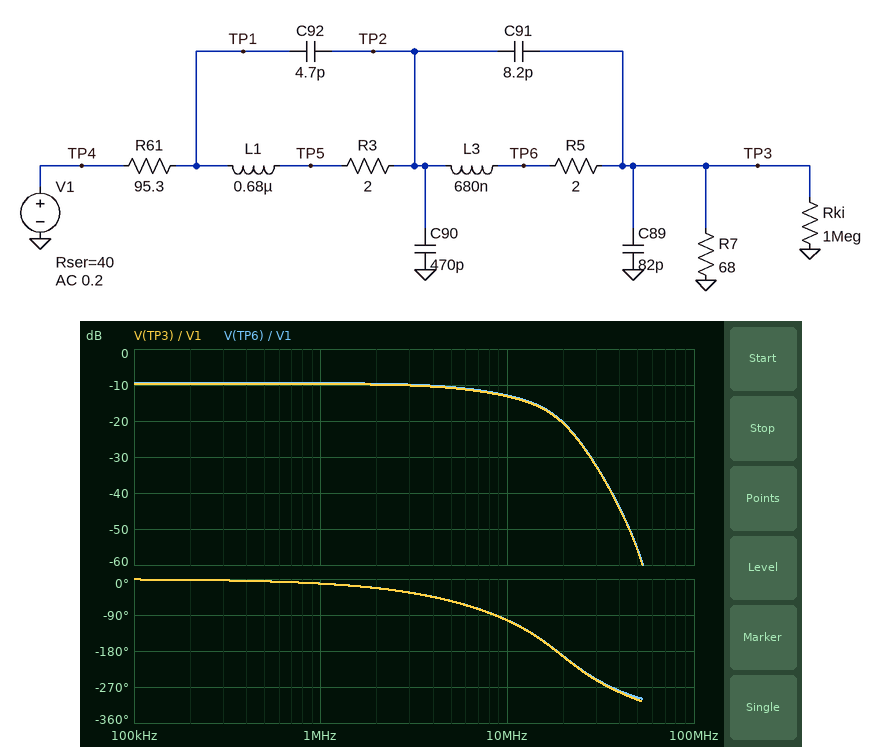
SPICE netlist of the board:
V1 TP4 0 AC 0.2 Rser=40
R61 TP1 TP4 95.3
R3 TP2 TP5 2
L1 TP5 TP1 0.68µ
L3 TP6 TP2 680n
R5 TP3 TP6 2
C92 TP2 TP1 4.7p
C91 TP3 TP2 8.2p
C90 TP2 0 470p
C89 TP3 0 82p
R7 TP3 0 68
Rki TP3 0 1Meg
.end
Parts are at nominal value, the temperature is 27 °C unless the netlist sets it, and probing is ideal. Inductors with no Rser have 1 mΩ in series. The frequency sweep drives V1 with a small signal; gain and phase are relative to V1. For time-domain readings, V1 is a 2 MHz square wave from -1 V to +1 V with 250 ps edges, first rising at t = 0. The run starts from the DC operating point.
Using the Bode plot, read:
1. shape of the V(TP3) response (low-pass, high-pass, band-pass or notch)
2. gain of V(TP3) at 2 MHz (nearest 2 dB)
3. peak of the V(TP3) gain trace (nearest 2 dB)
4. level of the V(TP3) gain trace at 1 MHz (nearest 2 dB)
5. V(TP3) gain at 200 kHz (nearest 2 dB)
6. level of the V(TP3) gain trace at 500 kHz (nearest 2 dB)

low-pass
-10 dB
-10 dB
-10 dB
-10 dB
-10 dB
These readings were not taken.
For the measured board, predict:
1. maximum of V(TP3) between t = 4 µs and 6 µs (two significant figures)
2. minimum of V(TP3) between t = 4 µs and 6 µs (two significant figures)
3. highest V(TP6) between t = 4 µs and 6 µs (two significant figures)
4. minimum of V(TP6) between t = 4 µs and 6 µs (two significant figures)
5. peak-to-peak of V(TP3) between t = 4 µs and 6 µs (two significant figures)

330 mV
-330 mV
340 mV
-340 mV
660 mV
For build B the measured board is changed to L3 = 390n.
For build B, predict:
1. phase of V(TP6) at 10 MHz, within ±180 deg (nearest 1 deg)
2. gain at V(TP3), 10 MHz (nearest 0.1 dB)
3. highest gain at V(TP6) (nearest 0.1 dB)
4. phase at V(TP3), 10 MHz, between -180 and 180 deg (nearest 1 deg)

-89 deg
-13.8 dB
-9.4 dB
-90 deg
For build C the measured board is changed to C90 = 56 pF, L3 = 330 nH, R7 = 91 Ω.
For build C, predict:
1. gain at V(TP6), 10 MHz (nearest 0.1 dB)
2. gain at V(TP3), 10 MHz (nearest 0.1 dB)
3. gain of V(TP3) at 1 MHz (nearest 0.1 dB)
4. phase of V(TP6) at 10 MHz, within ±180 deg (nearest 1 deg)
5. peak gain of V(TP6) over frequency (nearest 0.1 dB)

-8.3 dB
-8.5 dB
-8.1 dB
-43 deg
-7.9 dB
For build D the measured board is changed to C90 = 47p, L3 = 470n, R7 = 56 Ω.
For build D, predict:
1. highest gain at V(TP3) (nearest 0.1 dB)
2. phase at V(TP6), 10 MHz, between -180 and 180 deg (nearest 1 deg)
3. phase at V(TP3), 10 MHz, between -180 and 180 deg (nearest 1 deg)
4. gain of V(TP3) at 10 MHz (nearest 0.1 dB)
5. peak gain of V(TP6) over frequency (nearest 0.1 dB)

-10.5 dB
-39 deg
-40 deg
-11.2 dB
-10.1 dB
